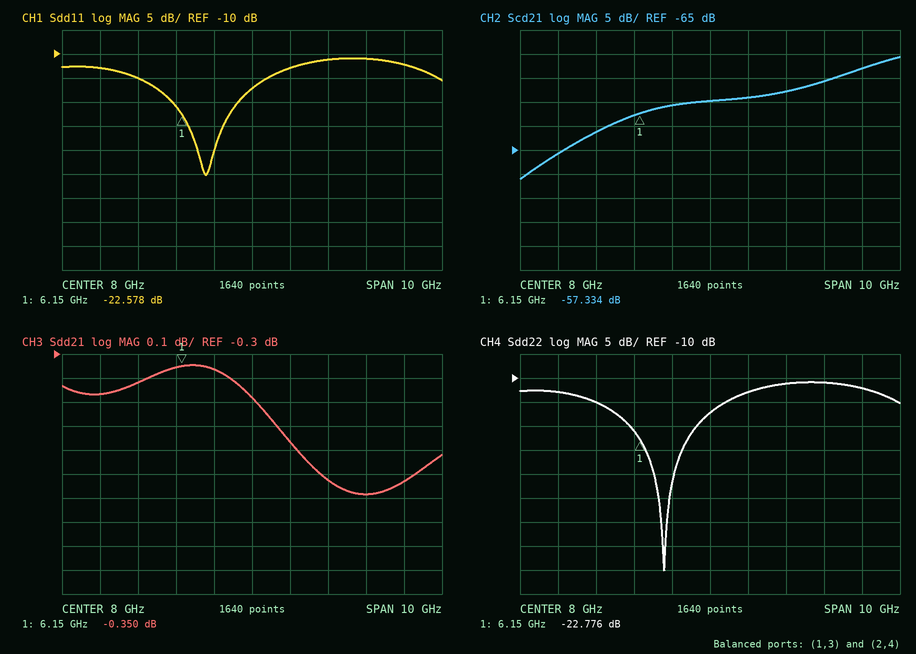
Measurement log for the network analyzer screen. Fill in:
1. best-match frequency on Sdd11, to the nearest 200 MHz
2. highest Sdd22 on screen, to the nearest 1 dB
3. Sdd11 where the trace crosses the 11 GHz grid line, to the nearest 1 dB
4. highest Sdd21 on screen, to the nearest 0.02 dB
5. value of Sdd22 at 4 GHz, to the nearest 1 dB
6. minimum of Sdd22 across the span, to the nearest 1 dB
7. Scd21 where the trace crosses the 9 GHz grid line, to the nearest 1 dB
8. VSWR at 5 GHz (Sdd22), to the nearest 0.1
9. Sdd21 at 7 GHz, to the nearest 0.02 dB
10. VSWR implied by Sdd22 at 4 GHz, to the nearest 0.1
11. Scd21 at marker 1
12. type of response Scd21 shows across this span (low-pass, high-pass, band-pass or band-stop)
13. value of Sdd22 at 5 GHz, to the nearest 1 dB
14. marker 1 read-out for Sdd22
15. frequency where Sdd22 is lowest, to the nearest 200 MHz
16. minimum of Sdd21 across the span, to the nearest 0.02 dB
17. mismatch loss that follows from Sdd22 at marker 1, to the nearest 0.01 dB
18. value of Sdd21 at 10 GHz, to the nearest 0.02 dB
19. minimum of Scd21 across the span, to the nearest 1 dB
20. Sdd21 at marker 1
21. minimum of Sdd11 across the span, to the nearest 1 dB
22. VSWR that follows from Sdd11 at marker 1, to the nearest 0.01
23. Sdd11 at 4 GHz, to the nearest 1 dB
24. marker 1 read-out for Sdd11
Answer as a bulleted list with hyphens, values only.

- 6.8 GHz
- -11 dB
- -11 dB
- -0.34 dB
- -13 dB
- -50 dB
- -54 dB
- 1.4
- -0.36 dB
- 1.6
- -57.334 dB
- high-pass
- -15 dB
- -22.776 dB
- 6.8 GHz
- -0.88 dB
- 0.02 dB
- -0.82 dB
- -71 dB
- -0.350 dB
- -35 dB
- 1.16
- -13 dB
- -22.578 dB
